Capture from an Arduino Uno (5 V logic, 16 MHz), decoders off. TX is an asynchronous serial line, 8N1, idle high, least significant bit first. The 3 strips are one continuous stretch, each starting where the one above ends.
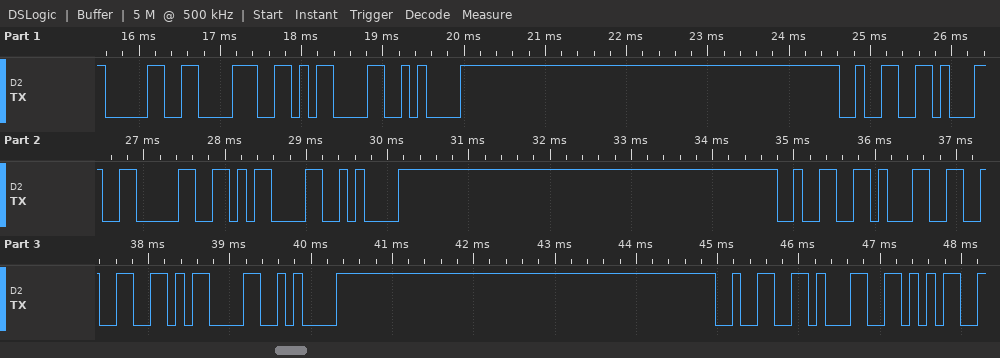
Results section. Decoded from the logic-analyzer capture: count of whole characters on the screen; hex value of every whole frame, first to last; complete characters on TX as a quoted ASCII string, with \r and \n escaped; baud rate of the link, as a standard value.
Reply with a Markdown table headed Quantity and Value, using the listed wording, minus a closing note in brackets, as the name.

| Quantity | Value |
|---|---|
| count of whole characters on the screen | 17 |
| hex value of every whole frame, first to last | 30 38 0D 0A 32 31 30 0D 0A 32 31 32 0D 0A 32 31 35 |
| complete characters on TX as a quoted ASCII string, with \r and \n escaped | "08\r\n210\r\n212\r\n215" |
| baud rate of the link, as a standard value | 9600 baud |
